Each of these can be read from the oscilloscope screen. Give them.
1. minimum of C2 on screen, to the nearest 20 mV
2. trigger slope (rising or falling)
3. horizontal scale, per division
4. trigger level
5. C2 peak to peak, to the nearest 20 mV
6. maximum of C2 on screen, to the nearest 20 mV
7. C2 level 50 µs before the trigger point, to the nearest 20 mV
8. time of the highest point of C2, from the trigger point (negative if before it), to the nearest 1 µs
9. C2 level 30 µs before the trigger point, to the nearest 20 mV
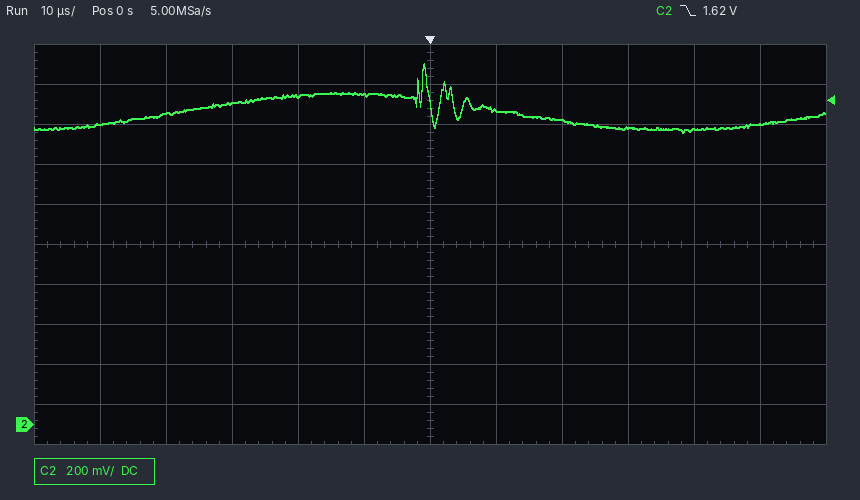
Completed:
1.46 V
falling
10 µs
1.62 V
340 mV
1.80 V
1.50 V
-1 µs
1.60 V
